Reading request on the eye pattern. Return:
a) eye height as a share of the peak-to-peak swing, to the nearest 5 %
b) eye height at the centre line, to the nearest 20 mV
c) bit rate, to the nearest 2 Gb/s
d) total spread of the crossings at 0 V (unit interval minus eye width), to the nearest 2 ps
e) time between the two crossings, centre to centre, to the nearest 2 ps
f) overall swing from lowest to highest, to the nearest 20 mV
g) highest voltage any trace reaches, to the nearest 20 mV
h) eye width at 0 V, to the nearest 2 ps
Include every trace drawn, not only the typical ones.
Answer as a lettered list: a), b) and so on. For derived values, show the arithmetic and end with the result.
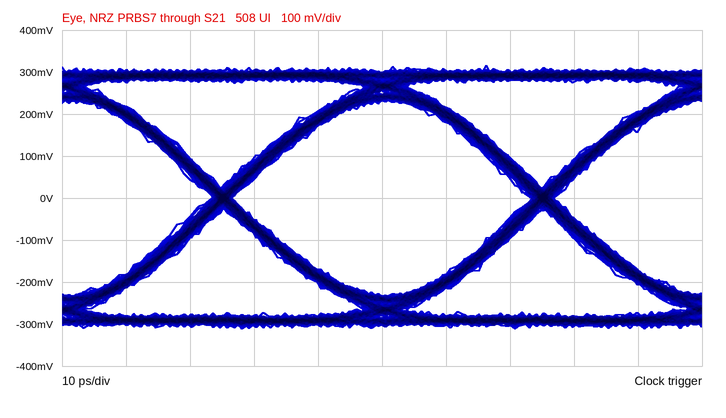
a) 460 mV / 620 mV ≈ 74.2 %, so 75 % to the nearest 5 %
b) 460 mV
c) 20 Gb/s
d) 4 ps
e) 50 ps
f) 620 mV
g) 320 mV
h) 46 ps
